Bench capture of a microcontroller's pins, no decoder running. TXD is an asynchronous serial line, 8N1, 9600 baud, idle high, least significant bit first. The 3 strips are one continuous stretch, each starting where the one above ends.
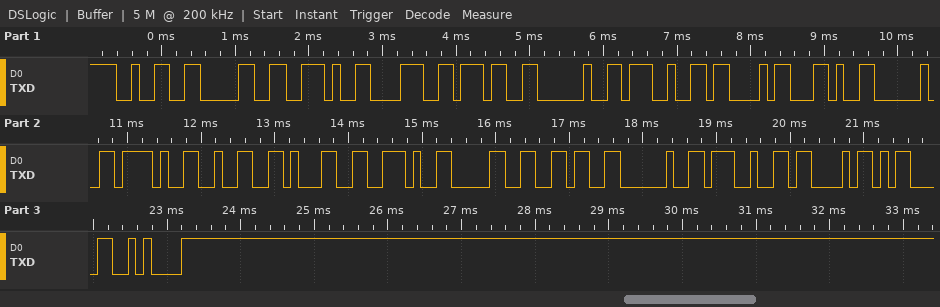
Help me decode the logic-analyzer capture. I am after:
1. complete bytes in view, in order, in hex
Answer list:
32 30 2E 38 37 20 27 43 2C 20 2F 32 31 2E 30 36 20 27 43 0D 0A
